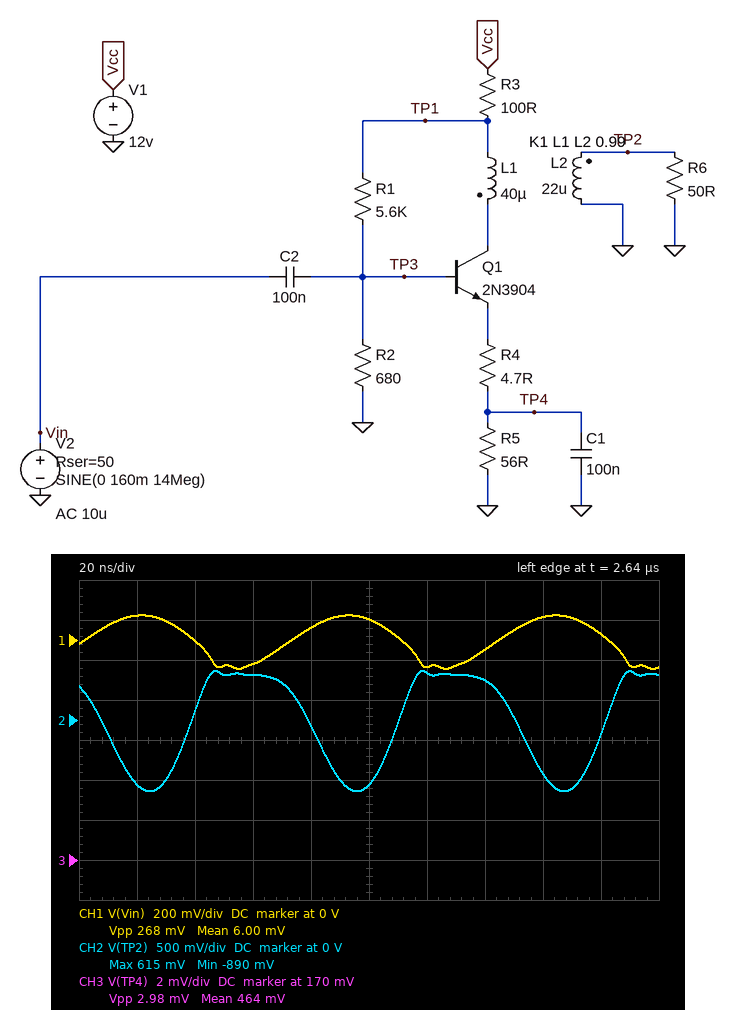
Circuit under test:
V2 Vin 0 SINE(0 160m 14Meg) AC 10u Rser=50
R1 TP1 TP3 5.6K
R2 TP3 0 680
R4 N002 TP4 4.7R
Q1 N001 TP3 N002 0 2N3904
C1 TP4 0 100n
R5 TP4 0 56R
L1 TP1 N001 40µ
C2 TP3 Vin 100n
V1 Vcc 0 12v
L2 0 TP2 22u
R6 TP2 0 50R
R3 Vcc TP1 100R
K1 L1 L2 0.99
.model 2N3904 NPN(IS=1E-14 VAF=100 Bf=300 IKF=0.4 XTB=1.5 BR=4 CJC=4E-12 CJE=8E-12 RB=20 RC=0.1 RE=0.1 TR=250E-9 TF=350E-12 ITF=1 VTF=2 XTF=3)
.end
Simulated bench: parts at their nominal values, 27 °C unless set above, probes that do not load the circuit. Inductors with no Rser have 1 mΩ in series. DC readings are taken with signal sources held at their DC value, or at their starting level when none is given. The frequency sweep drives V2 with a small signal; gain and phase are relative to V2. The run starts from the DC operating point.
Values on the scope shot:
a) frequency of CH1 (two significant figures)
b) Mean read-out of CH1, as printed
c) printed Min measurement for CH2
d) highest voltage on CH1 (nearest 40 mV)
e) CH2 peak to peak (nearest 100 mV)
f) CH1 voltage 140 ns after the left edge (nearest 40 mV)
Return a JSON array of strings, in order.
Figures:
["14 MHz", "6.00 mV", "-890 mV", "120 mV", "1.5 V", "-40 mV"]
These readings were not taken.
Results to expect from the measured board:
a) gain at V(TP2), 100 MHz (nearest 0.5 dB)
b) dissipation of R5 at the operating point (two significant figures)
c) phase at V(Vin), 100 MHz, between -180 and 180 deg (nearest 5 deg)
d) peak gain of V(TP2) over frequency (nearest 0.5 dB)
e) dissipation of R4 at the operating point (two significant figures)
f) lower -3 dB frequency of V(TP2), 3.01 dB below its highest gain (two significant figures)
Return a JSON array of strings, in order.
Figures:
["3.5 dB", "3.4 mW", "-15 deg", "16.5 dB", "290 µW", "440 kHz"]
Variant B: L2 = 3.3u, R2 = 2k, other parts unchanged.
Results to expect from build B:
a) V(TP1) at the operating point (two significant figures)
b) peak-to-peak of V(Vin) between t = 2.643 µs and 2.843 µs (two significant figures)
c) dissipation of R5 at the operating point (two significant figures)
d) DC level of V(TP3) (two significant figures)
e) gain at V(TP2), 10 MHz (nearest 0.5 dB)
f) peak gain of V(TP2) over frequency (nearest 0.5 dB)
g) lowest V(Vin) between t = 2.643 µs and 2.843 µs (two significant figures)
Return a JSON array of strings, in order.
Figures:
["9.3 V", "170 mV", "38 mW", "2.3 V", "25.0 dB", "27.0 dB", "-88 mV"]
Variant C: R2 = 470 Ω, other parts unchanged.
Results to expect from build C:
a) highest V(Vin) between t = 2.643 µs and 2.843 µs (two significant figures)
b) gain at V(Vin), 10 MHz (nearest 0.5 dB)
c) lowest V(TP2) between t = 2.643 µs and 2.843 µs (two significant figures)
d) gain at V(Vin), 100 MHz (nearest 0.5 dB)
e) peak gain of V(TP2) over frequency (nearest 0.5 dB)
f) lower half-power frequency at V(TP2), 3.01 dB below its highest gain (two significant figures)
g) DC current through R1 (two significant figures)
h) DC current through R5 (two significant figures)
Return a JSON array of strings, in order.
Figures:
["130 mV", "-1.5 dB", "-610 mV", "-11.5 dB", "13.0 dB", "410 kHz", "1.9 mA", "3.3 mA"]
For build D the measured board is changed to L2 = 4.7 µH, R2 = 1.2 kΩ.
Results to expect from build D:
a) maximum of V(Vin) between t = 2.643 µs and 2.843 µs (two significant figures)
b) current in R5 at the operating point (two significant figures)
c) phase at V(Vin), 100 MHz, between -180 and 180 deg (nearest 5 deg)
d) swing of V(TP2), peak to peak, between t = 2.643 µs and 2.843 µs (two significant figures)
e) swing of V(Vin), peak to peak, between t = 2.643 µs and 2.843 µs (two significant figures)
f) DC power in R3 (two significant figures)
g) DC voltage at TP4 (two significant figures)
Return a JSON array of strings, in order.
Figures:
["96 mV", "17 mA", "-10 deg", "4.0 V", "210 mV", "33 mW", "940 mV"]
